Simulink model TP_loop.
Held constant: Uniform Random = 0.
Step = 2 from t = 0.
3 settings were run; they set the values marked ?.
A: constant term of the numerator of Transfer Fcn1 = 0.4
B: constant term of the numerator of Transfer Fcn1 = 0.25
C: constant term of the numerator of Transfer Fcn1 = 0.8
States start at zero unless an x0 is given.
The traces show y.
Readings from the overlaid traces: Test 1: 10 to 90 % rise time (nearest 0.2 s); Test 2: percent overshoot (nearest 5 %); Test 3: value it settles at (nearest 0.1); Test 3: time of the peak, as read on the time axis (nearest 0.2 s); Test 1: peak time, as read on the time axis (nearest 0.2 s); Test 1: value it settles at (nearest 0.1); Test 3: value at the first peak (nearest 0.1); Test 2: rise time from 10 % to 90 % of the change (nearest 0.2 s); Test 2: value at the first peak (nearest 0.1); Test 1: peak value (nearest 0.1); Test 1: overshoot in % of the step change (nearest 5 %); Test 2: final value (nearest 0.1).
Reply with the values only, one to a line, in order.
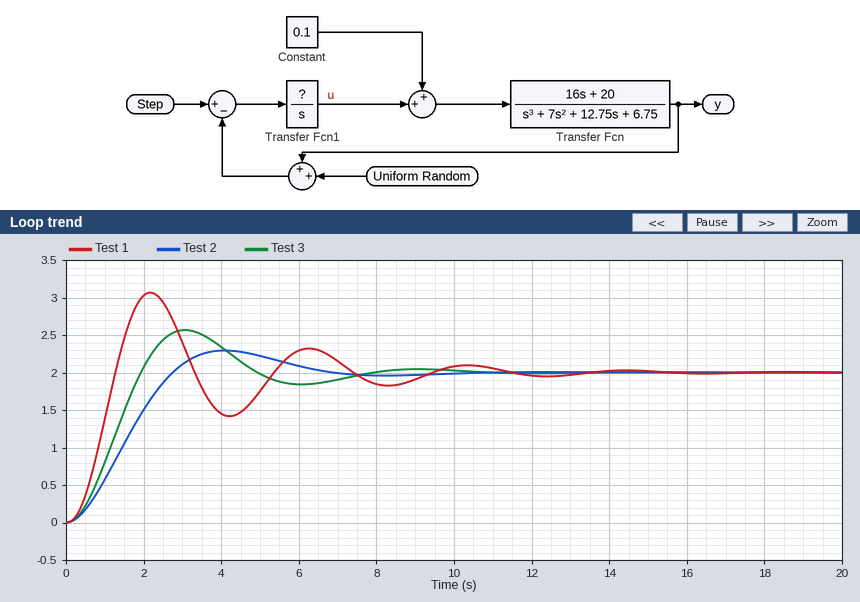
0.8 s
15 %
2.0
3.0 s
2.2 s
2.0
2.6
1.8 s
2.3
3.1
55 %
2.0
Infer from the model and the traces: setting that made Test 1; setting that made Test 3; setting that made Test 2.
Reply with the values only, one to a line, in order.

C
A
B
